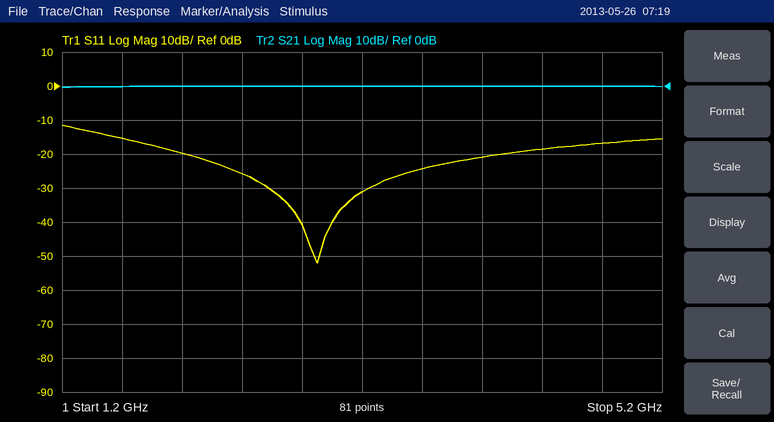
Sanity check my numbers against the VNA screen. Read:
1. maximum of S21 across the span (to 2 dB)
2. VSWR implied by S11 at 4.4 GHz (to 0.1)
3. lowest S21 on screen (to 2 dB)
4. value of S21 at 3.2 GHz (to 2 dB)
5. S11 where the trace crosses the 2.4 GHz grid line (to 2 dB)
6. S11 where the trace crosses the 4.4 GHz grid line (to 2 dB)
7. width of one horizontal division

0 dB
1.3
0 dB
0 dB
-26 dB
-18 dB
400 MHz
